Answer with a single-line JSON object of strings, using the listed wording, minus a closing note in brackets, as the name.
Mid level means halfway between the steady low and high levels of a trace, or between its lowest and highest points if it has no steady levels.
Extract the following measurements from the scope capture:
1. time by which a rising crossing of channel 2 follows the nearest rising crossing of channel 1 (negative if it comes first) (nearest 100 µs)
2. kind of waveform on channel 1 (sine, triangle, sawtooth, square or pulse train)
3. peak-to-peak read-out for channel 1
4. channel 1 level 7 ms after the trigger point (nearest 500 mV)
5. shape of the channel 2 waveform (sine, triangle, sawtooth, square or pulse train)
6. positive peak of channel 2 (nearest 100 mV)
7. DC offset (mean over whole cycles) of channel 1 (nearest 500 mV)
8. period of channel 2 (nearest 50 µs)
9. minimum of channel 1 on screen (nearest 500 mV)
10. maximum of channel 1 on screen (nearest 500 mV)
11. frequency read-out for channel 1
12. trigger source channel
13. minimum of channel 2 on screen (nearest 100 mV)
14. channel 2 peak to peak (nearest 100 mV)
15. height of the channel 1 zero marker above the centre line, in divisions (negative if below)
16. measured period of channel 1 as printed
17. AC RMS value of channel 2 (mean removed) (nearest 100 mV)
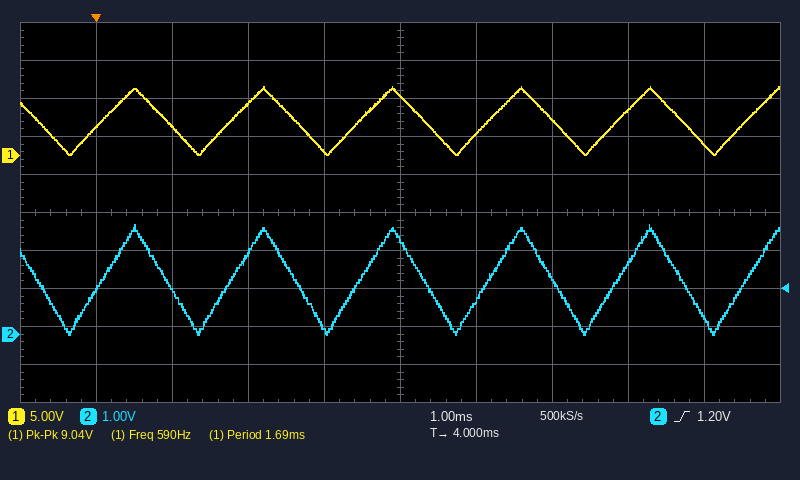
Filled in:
{"time by which a rising crossing of channel 2 follows the nearest rising crossing of channel 1 (negative if it comes first)": "0.0 ms", "kind of waveform on channel 1": "triangle", "peak-to-peak read-out for channel 1": "9.04 V", "channel 1 level 7 ms after the trigger point": "6.0 V", "shape of the channel 2 waveform": "triangle", "positive peak of channel 2": "2.9 V", "DC offset (mean over whole cycles) of channel 1": "4.5 V", "period of channel 2": "1.70 ms", "minimum of channel 1 on screen": "0.0 V", "maximum of channel 1 on screen": "9.0 V", "frequency read-out for channel 1": "590 Hz", "trigger source channel": "channel 2", "minimum of channel 2 on screen": "0.0 V", "channel 2 peak to peak": "2.9 V", "height of the channel 1 zero marker above the centre line, in divisions": "+1.5 div", "measured period of channel 1 as printed": "1.69 ms", "AC RMS value of channel 2 (mean removed)": "800 mV"}
